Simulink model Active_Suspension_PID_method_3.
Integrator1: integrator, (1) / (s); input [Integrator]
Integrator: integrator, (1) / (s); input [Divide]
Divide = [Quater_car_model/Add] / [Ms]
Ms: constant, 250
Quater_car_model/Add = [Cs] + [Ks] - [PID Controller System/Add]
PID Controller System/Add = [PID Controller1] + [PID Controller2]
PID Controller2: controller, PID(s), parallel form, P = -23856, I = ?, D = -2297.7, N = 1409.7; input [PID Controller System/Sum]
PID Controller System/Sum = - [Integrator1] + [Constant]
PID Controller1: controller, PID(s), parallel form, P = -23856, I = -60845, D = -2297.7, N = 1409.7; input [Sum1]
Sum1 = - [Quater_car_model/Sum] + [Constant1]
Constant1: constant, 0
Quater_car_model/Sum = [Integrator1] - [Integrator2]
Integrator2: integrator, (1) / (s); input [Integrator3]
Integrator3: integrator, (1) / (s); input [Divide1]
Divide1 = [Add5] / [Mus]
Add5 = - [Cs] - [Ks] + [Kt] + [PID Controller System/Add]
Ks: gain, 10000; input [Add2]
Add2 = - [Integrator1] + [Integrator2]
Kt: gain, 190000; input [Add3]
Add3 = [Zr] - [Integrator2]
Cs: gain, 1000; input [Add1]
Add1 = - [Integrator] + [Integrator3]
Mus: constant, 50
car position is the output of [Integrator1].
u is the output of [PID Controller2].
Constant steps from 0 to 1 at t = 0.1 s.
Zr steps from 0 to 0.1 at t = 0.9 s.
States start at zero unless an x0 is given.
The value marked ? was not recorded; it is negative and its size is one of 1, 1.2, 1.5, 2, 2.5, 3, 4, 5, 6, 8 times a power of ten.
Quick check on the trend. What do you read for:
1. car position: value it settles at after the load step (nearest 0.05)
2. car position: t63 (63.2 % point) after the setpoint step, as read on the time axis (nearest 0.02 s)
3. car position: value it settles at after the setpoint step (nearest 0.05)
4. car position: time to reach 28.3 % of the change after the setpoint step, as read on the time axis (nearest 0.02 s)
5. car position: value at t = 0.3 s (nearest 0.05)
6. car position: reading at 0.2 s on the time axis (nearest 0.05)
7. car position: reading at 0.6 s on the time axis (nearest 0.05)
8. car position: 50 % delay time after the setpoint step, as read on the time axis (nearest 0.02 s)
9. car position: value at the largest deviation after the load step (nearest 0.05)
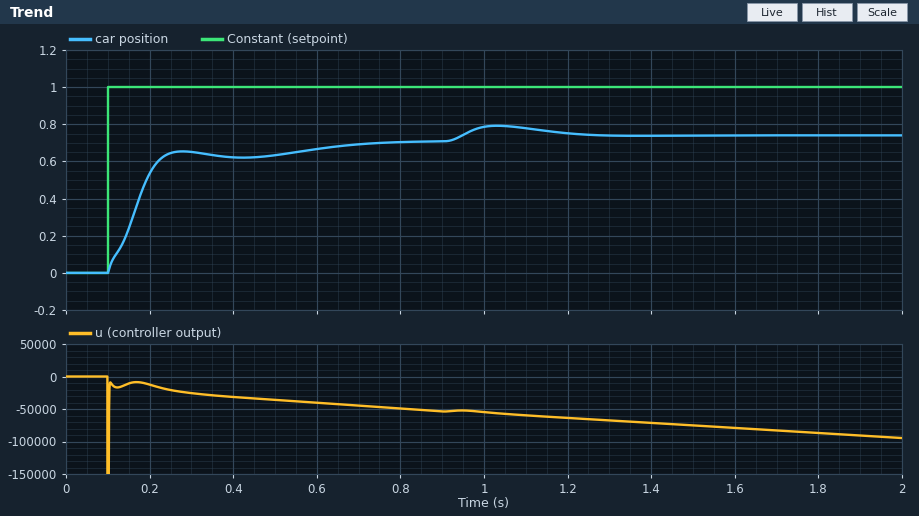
0.75
0.18 s
0.70
0.14 s
0.65
0.55
0.65
0.16 s
0.80
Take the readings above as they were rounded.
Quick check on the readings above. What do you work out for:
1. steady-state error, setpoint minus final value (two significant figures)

0.30
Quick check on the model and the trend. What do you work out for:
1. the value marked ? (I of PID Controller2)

-150000
